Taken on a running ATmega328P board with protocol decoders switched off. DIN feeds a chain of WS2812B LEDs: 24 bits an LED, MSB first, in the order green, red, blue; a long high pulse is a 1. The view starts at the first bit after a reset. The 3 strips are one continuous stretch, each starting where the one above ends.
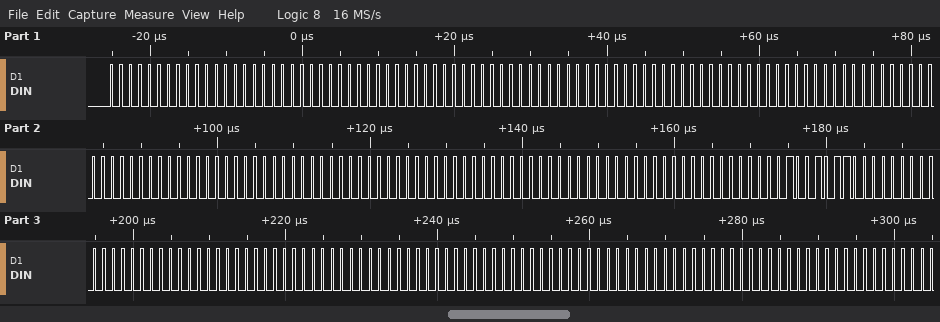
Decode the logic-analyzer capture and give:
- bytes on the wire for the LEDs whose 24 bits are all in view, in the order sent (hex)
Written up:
00 00 00 00 00 00 00 00 00 00 00 00 00 00 00 00 00 00 00 00 96 00 00 00 00 00 00 00 00 00 00 00 00
